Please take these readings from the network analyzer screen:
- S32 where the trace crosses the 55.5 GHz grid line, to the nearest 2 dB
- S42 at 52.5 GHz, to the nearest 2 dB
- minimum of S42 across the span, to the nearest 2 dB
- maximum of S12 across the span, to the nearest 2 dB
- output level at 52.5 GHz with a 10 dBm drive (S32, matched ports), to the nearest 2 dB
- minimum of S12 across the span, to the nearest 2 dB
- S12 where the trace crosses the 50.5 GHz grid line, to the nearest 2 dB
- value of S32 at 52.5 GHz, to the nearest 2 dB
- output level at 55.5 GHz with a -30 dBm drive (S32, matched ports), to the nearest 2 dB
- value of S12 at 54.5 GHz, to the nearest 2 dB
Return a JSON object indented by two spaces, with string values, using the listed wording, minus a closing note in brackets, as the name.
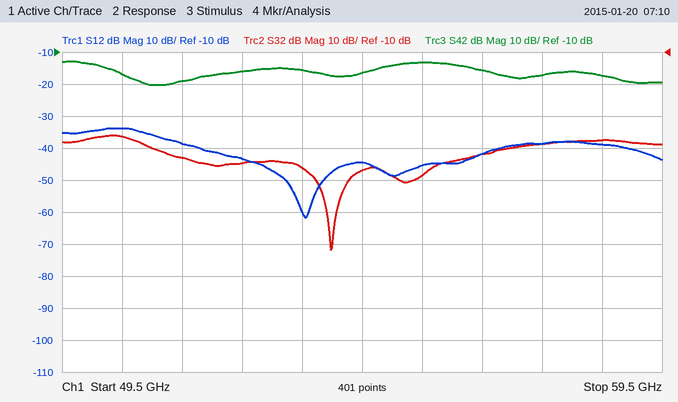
{
  "S32 where the trace crosses the 55.5 GHz grid line, to the nearest 2 dB": "-48 dB",
  "S42 at 52.5 GHz, to the nearest 2 dB": "-16 dB",
  "minimum of S42 across the span, to the nearest 2 dB": "-20 dB",
  "maximum of S12 across the span, to the nearest 2 dB": "-34 dB",
  "output level at 52.5 GHz with a 10 dBm drive (S32, matched ports), to the nearest 2 dB": "-34 dBm",
  "minimum of S12 across the span, to the nearest 2 dB": "-62 dB",
  "S12 where the trace crosses the 50.5 GHz grid line, to the nearest 2 dB": "-34 dB",
  "value of S32 at 52.5 GHz, to the nearest 2 dB": "-44 dB",
  "output level at 55.5 GHz with a -30 dBm drive (S32, matched ports), to the nearest 2 dB": "-78 dBm",
  "value of S12 at 54.5 GHz, to the nearest 2 dB": "-44 dB"
}
